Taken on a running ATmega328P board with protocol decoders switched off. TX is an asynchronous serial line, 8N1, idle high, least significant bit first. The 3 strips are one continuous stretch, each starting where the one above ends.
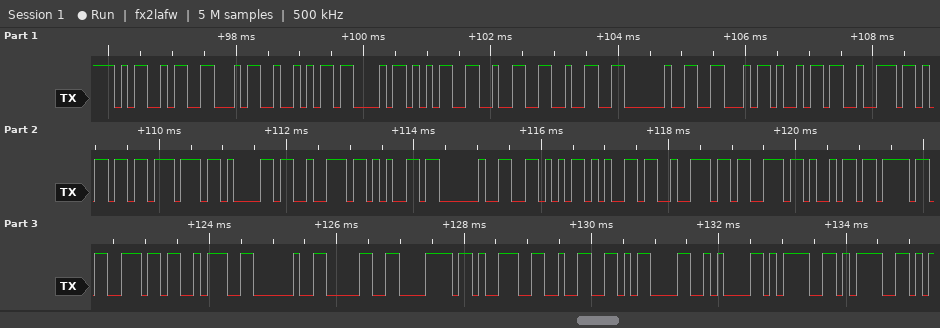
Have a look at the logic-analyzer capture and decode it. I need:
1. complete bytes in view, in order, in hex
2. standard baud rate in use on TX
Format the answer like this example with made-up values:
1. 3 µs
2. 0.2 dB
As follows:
1. 0x4D 0x46 0x52 0x43 0x35 0x32 0x32 0x20 0x46 0x69 0x72 0x6D 0x77 0x61 0x72 0x65 0x20 0x56 0x65 0x72 0x73 0x69 0x6F 0x6E 0x3A 0x20 0x30 0x78 0x39 0x32 0x0D 0x0A 0x3D 0x3D
2. 9600 baud
